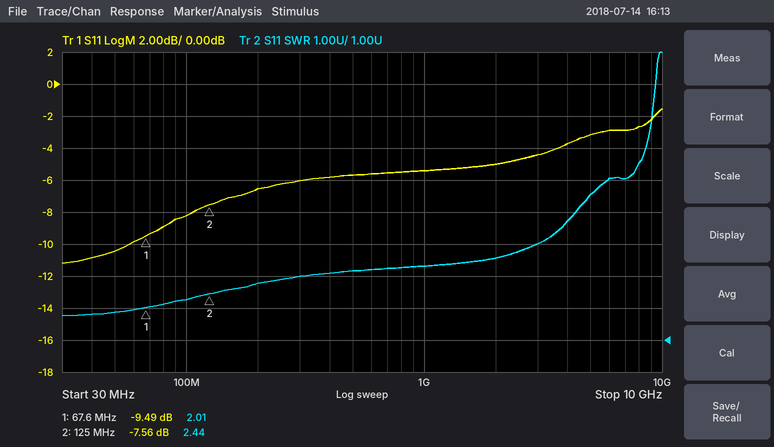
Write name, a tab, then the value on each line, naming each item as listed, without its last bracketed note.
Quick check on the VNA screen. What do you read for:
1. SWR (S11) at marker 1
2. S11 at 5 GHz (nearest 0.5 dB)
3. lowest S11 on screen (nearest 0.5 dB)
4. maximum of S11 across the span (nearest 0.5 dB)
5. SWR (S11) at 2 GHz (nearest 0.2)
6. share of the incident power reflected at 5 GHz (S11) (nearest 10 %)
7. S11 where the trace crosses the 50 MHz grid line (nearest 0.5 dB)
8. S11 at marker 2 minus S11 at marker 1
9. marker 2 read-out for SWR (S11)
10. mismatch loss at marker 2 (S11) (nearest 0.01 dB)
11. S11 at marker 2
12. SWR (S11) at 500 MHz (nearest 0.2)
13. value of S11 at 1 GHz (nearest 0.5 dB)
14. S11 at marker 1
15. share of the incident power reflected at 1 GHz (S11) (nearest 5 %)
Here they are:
SWR (S11) at marker 1	2.01
S11 at 5 GHz	-3.0 dB
lowest S11 on screen	-11.0 dB
maximum of S11 across the span	-1.5 dB
SWR (S11) at 2 GHz	3.6
share of the incident power reflected at 5 GHz (S11)	50 %
S11 where the trace crosses the 50 MHz grid line	-10.5 dB
S11 at marker 2 minus S11 at marker 1	1.93 dB
marker 2 read-out for SWR	2.44
mismatch loss at marker 2 (S11)	0.84 dB
S11 at marker 2	-7.56 dB
SWR (S11) at 500 MHz	3.2
value of S11 at 1 GHz	-5.5 dB
S11 at marker 1	-9.49 dB
share of the incident power reflected at 1 GHz (S11)	30 %
